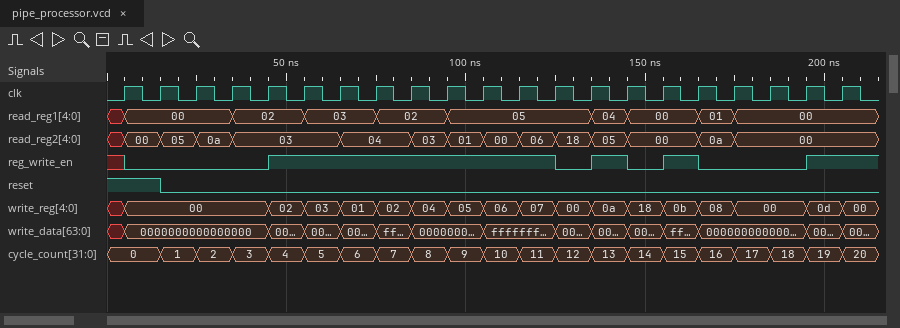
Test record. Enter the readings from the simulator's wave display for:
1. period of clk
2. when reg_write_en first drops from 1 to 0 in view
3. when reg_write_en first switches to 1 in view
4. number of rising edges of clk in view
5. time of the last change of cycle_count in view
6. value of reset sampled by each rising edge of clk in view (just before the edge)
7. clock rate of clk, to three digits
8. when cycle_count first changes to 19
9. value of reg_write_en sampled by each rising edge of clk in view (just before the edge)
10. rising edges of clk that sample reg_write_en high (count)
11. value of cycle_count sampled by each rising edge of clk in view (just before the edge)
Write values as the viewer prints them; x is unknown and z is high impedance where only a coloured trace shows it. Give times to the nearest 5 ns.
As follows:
10 ns
125 ns
45 ns
21
205 ns
1 1 0 0 0 0 0 0 0 0 0 0 0 0 0 0 0 0 0 0 0
100 MHz
195 ns
x 0 0 0 0 1 1 1 1 1 1 1 1 0 1 0 1 0 0 0 1
11
0, 0, 1, 2, 3, 4, 5, 6, 7, 8, 9, 10, 11, 12, 13, 14, 15, 16, 17, 18, 19
